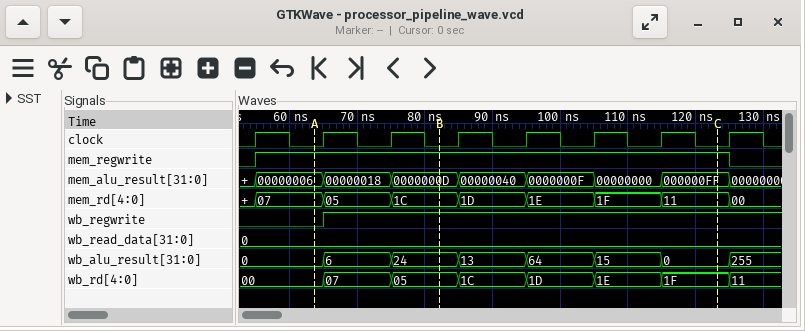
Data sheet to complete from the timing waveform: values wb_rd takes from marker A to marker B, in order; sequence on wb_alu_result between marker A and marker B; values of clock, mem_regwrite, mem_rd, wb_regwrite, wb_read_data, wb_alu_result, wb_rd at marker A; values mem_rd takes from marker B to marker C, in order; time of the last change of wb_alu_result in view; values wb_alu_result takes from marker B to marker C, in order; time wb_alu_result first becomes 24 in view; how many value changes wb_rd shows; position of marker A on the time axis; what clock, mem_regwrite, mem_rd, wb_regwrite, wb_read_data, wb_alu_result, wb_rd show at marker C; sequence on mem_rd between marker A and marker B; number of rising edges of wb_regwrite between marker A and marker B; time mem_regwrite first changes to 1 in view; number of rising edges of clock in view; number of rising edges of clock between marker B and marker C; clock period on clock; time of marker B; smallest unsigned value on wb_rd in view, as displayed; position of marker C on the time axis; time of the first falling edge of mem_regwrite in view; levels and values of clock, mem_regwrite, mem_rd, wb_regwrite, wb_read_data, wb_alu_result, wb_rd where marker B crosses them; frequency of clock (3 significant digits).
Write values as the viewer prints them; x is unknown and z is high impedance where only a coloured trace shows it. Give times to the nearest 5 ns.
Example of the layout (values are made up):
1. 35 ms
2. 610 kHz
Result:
1. 00, 07, 05
2. 0, 6, 24
3. clock=0, mem_regwrite=1, mem_rd=07, wb_regwrite=0, wb_read_data=0, wb_alu_result=0, wb_rd=00
4. 1C, 1D, 1E, 1F, 11
5. 125 ns
6. 24, 13, 64, 15, 0
7. 75 ns
8. 7
9. 65 ns
10. clock=0, mem_regwrite=1, mem_rd=11, wb_regwrite=1, wb_read_data=0, wb_alu_result=0, wb_rd=1F
11. 07, 05, 1C
12. 1
13. 55 ns
14. 8
15. 4
16. 10 ns
17. 80 ns
18. 00
19. 125 ns
20. 125 ns
21. clock=0, mem_regwrite=1, mem_rd=1C, wb_regwrite=1, wb_read_data=0, wb_alu_result=24, wb_rd=05
22. 100 MHz
